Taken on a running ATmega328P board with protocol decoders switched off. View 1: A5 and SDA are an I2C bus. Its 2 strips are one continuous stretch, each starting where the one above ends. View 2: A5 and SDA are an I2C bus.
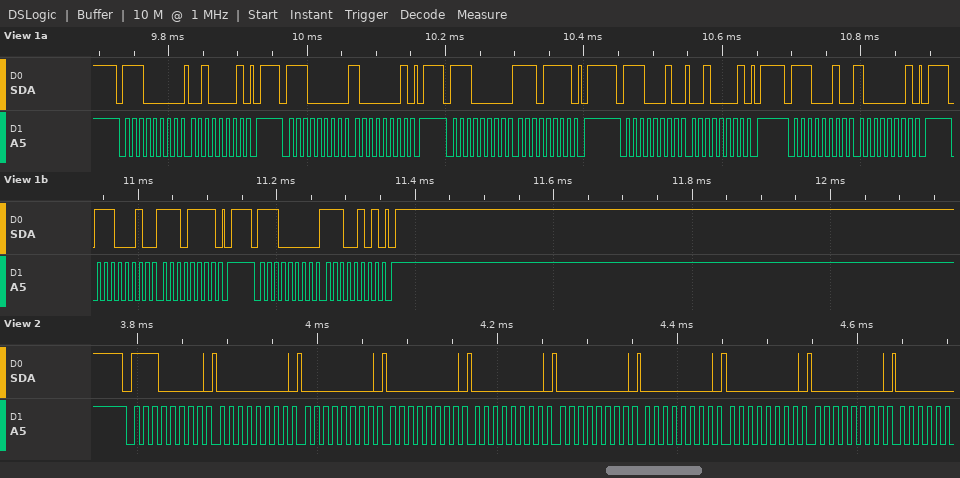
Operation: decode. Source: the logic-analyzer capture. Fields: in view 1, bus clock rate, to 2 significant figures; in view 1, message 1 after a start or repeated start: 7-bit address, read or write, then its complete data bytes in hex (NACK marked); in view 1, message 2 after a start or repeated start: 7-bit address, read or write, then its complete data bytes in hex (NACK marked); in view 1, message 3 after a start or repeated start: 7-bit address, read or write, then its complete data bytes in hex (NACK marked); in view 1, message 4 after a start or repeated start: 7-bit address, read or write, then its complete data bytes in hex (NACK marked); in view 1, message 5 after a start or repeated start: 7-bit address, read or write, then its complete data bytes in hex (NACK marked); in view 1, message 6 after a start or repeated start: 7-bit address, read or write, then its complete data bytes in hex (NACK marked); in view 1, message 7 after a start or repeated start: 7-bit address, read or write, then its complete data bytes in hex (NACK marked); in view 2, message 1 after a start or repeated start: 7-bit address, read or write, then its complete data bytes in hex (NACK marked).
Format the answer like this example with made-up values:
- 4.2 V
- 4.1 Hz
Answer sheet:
- 100 kHz
- 0x70 write: 21
- 0x70 write: 81
- 0x70 write: EF
- 0x71 write: 21
- 0x71 write: 81
- 0x71 write: EF
- 0x70 write: E5
- 0x70 write: 00 00 00 00 00 00 00 00
